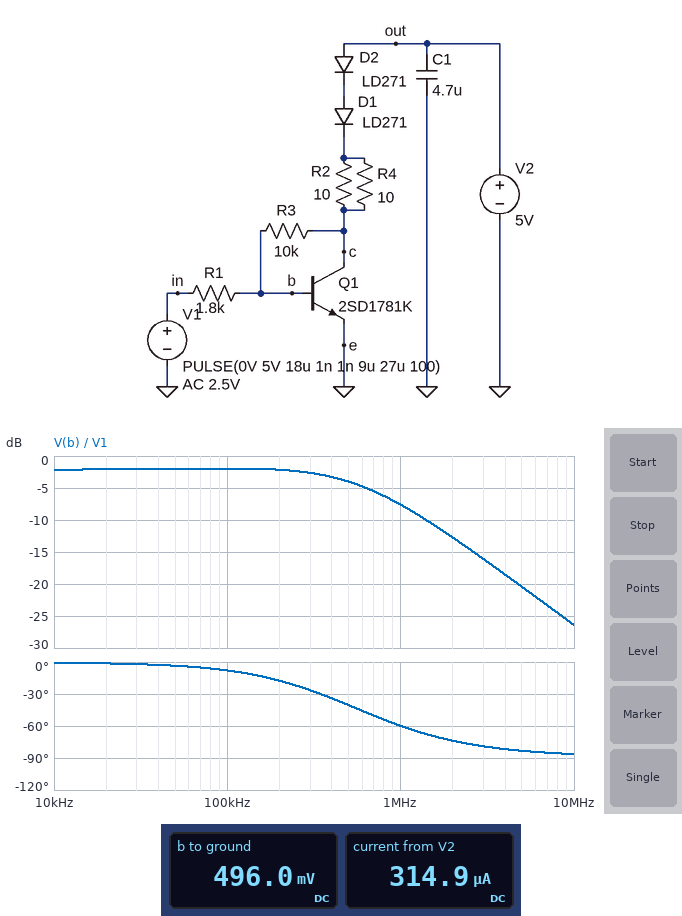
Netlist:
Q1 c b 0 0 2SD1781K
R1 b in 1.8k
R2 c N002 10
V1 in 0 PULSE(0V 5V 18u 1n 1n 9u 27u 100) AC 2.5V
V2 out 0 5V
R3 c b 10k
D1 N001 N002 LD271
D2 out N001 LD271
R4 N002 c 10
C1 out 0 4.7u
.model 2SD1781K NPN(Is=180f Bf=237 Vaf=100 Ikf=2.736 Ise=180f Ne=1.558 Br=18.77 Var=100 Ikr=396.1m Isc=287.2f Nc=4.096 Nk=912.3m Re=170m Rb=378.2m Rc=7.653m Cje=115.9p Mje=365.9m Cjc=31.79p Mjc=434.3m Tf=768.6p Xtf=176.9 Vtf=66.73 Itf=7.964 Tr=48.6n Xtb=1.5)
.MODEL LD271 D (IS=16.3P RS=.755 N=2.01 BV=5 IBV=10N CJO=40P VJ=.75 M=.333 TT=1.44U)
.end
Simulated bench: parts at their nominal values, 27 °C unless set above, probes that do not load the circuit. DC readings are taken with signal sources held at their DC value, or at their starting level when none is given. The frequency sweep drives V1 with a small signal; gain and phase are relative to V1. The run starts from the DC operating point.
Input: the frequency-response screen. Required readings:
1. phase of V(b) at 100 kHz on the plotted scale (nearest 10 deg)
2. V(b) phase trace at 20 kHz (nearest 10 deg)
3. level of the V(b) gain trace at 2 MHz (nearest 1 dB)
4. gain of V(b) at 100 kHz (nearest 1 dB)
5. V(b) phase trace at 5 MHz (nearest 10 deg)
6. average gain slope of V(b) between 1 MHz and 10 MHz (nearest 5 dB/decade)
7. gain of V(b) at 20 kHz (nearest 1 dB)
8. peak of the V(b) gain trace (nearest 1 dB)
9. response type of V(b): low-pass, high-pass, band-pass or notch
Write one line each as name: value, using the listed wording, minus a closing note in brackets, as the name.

phase of V(b) at 100 kHz on the plotted scale: -10 deg
V(b) phase trace at 20 kHz: 0 deg
level of the V(b) gain trace at 2 MHz: -13 dB
gain of V(b) at 100 kHz: -2 dB
V(b) phase trace at 5 MHz: -80 deg
average gain slope of V(b) between 1 MHz and 10 MHz: -20 dB/decade
gain of V(b) at 20 kHz: -2 dB
peak of the V(b) gain trace: -2 dB
response type of V(b): low-pass, high-pass, band-pass or notch: low-pass
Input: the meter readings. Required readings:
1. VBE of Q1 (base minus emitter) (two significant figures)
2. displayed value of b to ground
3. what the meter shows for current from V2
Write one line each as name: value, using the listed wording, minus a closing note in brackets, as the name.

VBE of Q1 (base minus emitter): 500 mV
displayed value of b to ground: 496.0 mV
what the meter shows for current from V2: 314.9 µA
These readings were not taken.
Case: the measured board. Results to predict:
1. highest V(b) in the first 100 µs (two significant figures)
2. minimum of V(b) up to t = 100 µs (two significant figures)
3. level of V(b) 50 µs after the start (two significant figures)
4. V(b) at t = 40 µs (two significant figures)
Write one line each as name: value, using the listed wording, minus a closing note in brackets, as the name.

highest V(b) in the first 100 µs: 800 mV
minimum of V(b) up to t = 100 µs: 400 mV
level of V(b) 50 µs after the start: 800 mV
V(b) at t = 40 µs: 490 mV
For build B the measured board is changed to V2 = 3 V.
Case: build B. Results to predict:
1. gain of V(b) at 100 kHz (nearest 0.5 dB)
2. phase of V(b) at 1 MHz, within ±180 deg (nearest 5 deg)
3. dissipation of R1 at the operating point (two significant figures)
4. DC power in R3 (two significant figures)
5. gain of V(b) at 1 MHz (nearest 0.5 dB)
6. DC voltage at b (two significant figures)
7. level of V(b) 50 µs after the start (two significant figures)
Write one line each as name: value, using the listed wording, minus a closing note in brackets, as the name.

gain of V(b) at 100 kHz: -1.5 dB
phase of V(b) at 1 MHz, within ±180 deg: -55 deg
dissipation of R1 at the operating point: 24 µW
DC power in R3: 130 µW
gain of V(b) at 1 MHz: -6.5 dB
DC voltage at b: 210 mV
level of V(b) 50 µs after the start: 730 mV
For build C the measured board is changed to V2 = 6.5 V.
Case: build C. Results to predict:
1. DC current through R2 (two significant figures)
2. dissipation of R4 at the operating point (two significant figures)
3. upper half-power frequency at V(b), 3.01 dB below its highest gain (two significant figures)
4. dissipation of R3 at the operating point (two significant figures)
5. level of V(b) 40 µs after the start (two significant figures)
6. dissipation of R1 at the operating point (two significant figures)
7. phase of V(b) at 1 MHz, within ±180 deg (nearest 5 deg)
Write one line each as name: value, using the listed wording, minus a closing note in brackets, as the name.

DC current through R2: 3.4 mA
dissipation of R4 at the operating point: 110 µW
upper half-power frequency at V(b), 3.01 dB below its highest gain: 840 kHz
dissipation of R3 at the operating point: 1.4 mW
level of V(b) 40 µs after the start: 630 mV
dissipation of R1 at the operating point: 220 µW
phase of V(b) at 1 MHz, within ±180 deg: -55 deg
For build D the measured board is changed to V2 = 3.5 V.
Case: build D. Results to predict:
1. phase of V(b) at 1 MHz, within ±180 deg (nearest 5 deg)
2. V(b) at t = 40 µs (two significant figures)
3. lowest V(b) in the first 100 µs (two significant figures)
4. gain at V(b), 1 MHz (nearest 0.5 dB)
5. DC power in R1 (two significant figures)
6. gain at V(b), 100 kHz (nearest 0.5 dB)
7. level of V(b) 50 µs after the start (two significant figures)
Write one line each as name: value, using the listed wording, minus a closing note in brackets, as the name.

phase of V(b) at 1 MHz, within ±180 deg: -55 deg
V(b) at t = 40 µs: 280 mV
lowest V(b) in the first 100 µs: 190 mV
gain at V(b), 1 MHz: -6.5 dB
DC power in R1: 43 µW
gain at V(b), 100 kHz: -1.5 dB
level of V(b) 50 µs after the start: 750 mV
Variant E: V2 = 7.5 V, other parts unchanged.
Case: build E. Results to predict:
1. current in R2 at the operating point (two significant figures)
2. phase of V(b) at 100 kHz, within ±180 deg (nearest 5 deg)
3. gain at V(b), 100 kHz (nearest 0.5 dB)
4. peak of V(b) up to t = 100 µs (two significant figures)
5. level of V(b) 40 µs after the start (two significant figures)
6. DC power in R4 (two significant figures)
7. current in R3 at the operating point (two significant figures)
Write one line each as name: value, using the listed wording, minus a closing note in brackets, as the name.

current in R2 at the operating point: 10 mA
phase of V(b) at 100 kHz, within ±180 deg: -5 deg
gain at V(b), 100 kHz: -17.5 dB
peak of V(b) up to t = 100 µs: 820 mV
level of V(b) 40 µs after the start: 660 mV
DC power in R4: 1.1 mW
current in R3 at the operating point: 450 µA
